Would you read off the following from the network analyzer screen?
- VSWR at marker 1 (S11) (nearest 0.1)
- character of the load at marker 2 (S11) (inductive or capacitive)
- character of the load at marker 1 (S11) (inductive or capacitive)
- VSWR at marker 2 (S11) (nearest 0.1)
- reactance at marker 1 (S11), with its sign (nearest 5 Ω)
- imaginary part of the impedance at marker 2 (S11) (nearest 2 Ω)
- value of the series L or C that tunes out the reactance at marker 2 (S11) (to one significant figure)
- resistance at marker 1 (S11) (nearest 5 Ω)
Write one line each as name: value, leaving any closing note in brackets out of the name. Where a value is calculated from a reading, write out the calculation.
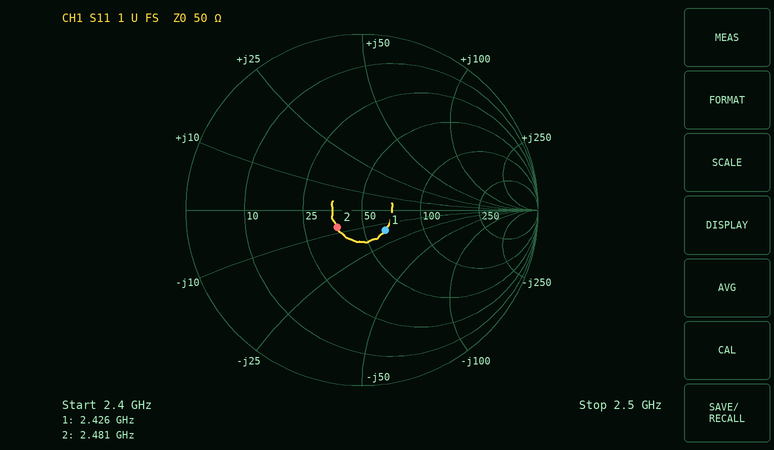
VSWR at marker 1 (S11): 1.4
character of the load at marker 2 (S11): capacitive
character of the load at marker 1 (S11): capacitive
VSWR at marker 2 (S11): 1.4
reactance at marker 1 (S11), with its sign: -15 Ω
imaginary part of the impedance at marker 2 (S11): -8 Ω
value of the series L or C that tunes out the reactance at marker 2 (S11): L = 8 Ω/(2π × 2.481 GHz) ≈ 513 pH, so 500 pH to one significant figure
resistance at marker 1 (S11): 65 Ω
